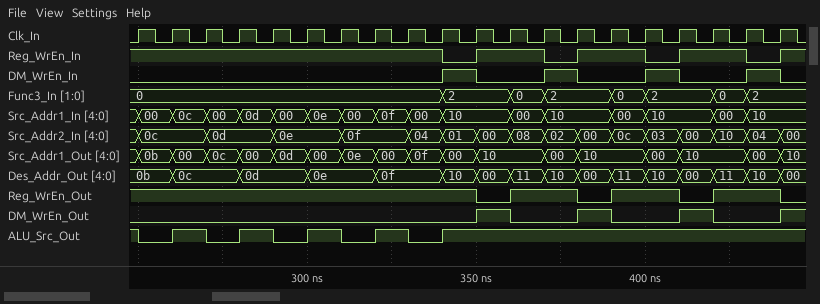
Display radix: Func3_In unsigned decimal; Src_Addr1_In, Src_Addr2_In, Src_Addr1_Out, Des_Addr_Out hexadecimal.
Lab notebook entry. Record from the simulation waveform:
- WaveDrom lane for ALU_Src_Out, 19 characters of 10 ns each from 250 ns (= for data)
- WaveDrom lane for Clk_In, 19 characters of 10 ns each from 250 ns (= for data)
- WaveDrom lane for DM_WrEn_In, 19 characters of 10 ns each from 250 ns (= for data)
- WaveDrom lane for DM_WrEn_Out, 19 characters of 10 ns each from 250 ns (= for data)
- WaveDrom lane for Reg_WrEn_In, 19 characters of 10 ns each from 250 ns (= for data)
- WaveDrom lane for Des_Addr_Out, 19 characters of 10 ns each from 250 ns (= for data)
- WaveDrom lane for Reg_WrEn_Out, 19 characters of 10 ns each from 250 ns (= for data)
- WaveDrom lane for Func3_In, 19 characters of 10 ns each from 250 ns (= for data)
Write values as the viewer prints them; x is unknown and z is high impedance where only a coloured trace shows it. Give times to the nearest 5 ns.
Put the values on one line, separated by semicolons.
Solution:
{name: 'ALU_Src_Out', wave: '0101010101.........'}; {name: 'Clk_In', wave: 'p..................'}; {name: 'DM_WrEn_In', wave: '0........10.10.10.1'}; {name: 'DM_WrEn_Out', wave: '0.........10.10.10.'}; {name: 'Reg_WrEn_In', wave: '1........01.01.01.0'}; {name: 'Des_Addr_Out', wave: '==.=.=.=.==========', data: '0b 0c 0d 0e 0f 10 00 11 10 00 11 10 00 11 10'}; {name: 'Reg_WrEn_Out', wave: '1.........01.01.01.'}; {name: 'Func3_In', wave: '=........=.==.==.==', data: '0 2 0 2 0 2 0 2'}
